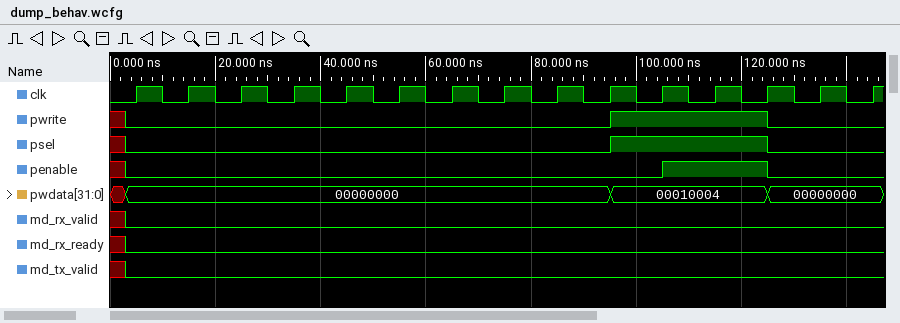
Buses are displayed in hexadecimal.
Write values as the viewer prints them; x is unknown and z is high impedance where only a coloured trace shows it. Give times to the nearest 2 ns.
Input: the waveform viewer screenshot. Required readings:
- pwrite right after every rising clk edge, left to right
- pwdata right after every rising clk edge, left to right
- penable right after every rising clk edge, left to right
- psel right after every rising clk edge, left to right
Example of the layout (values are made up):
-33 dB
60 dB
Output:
0 0 0 0 0 0 0 0 0 1 1 1 0 0 0
00000000, 00000000, 00000000, 00000000, 00000000, 00000000, 00000000, 00000000, 00000000, 00010004, 00010004, 00010004, 00000000, 00000000, 00000000
0 0 0 0 0 0 0 0 0 0 1 1 0 0 0
0 0 0 0 0 0 0 0 0 1 1 1 0 0 0
